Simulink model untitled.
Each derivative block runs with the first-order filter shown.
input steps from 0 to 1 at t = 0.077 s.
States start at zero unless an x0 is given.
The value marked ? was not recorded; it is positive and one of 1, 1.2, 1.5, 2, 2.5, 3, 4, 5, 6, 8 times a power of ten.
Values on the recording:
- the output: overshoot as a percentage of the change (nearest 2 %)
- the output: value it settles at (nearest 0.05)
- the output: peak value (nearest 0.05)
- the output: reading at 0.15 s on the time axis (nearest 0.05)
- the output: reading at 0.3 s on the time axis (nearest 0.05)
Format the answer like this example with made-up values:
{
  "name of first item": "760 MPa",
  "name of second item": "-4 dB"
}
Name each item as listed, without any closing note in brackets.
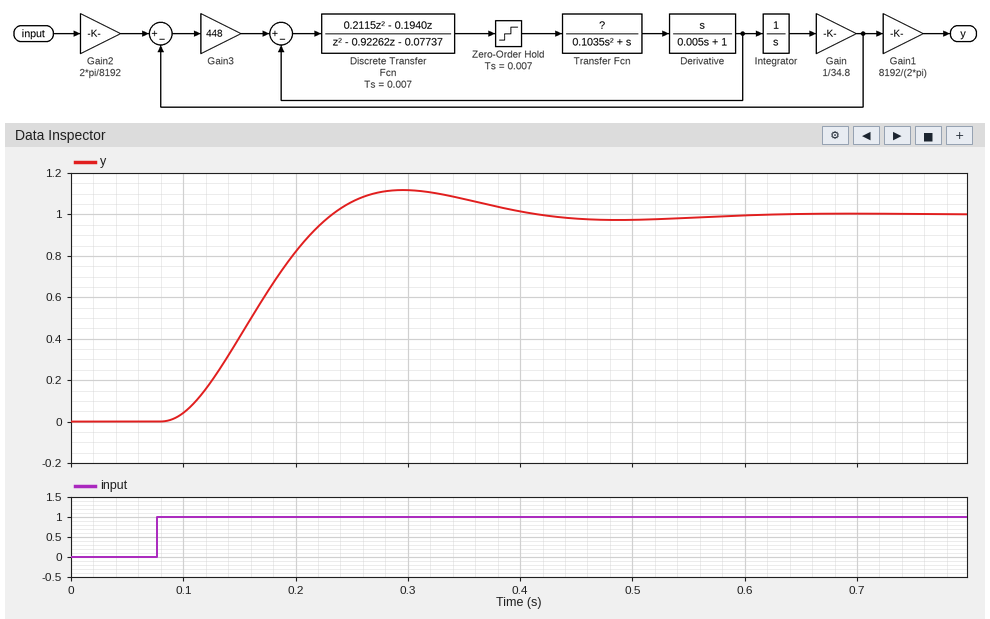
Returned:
{
  "the output: overshoot as a percentage of the change": "12 %",
  "the output: value it settles at": "1.00",
  "the output: peak value": "1.10",
  "the output: reading at 0.15 s on the time axis": "0.40",
  "the output: reading at 0.3 s on the time axis": "1.10"
}
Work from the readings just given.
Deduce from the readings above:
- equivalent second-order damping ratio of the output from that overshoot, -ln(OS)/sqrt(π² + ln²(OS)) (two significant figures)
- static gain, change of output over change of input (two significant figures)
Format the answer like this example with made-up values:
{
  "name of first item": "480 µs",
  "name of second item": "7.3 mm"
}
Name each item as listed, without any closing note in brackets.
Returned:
{
  "equivalent second-order damping ratio of the output from that overshoot, -ln(OS)/sqrt(π² + ln²(OS))": "0.56",
  "static gain, change of output over change of input": "1.0"
}
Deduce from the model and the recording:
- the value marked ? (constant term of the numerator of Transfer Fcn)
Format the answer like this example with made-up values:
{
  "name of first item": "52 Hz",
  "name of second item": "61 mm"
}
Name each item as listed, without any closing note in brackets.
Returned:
{
  "the value marked ?": "10"
}
